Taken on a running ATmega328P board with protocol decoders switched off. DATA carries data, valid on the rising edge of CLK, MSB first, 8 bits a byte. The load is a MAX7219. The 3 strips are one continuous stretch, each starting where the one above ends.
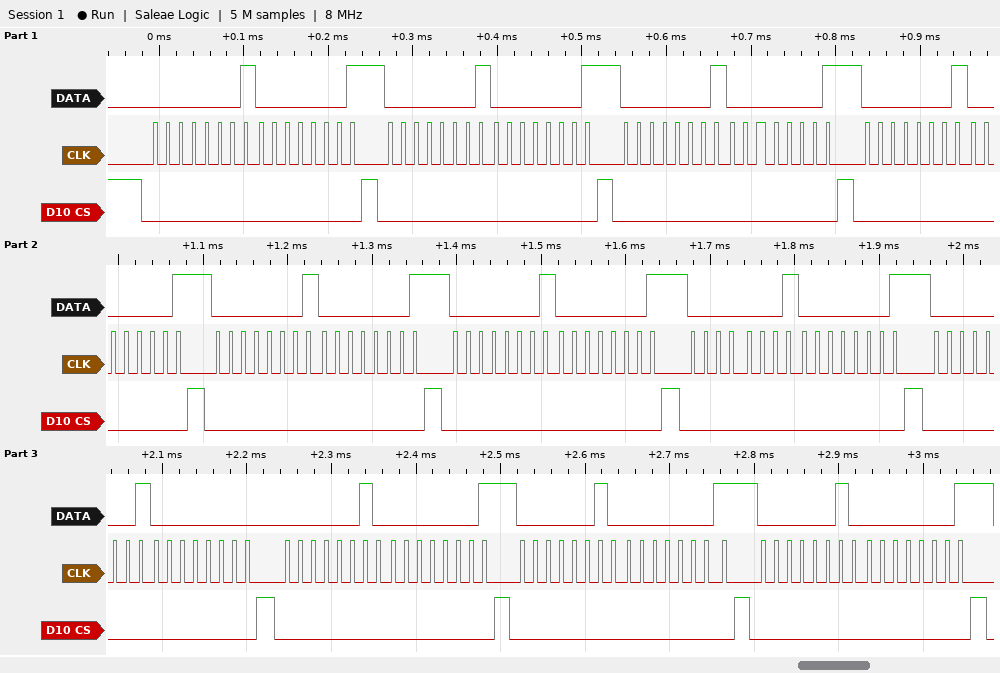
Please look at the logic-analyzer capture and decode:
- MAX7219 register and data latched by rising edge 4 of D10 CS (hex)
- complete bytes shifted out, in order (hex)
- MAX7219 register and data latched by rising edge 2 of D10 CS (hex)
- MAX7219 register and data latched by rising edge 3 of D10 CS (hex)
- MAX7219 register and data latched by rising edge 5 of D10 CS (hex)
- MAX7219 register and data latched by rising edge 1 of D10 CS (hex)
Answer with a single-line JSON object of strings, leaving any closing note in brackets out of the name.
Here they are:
{"MAX7219 register and data latched by rising edge 4 of D10 CS": "register 0x1, data 0x01", "complete bytes shifted out, in order": "01 01 01 01 01 01 01 01 01 01 01 01 01 01 01 00 02 01 02 01 02 01", "MAX7219 register and data latched by rising edge 2 of D10 CS": "register 0x1, data 0x01", "MAX7219 register and data latched by rising edge 3 of D10 CS": "register 0x1, data 0x01", "MAX7219 register and data latched by rising edge 5 of D10 CS": "register 0x1, data 0x01", "MAX7219 register and data latched by rising edge 1 of D10 CS": "register 0x1, data 0x01"}
